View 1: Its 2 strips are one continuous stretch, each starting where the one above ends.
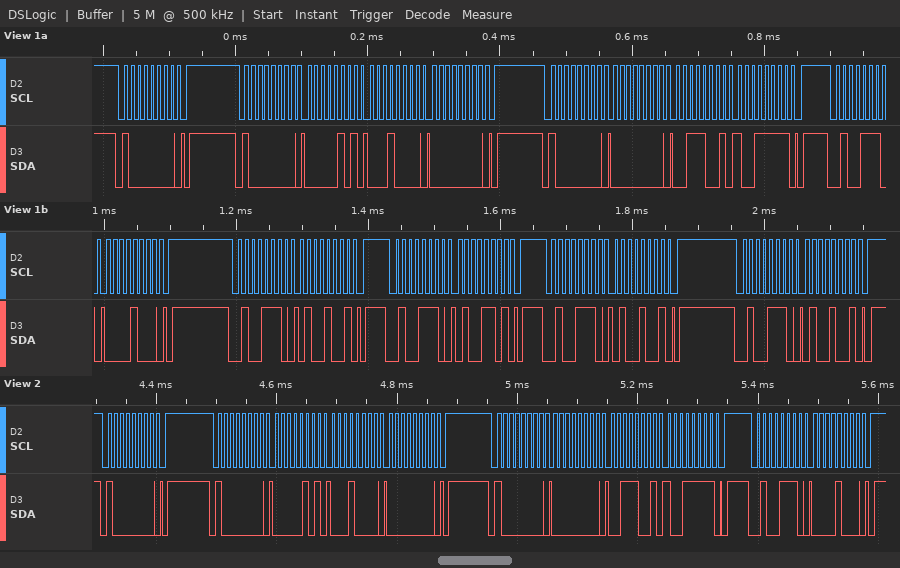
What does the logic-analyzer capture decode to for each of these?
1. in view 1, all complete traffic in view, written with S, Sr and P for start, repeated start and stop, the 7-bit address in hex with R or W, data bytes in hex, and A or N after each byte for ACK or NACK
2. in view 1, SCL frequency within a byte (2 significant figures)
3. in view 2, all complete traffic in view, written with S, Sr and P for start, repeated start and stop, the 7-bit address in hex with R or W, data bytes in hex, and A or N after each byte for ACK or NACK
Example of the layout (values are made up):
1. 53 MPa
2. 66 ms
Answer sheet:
1. S 40W A P S 40W A 05 A 10 A 00 A P S 40W A 00 A 39 A 9F A P S 27W A 08 A P S 27W A 49 A P S 27W A 4D A P S 27W A 49 A P S 27W A 49 A P
2. 100 kHz
3. S 40W A P S 40W A 05 A 10 A 00 A P S 40W A 00 A 39 A 9F A P S 27W A 08 A P
